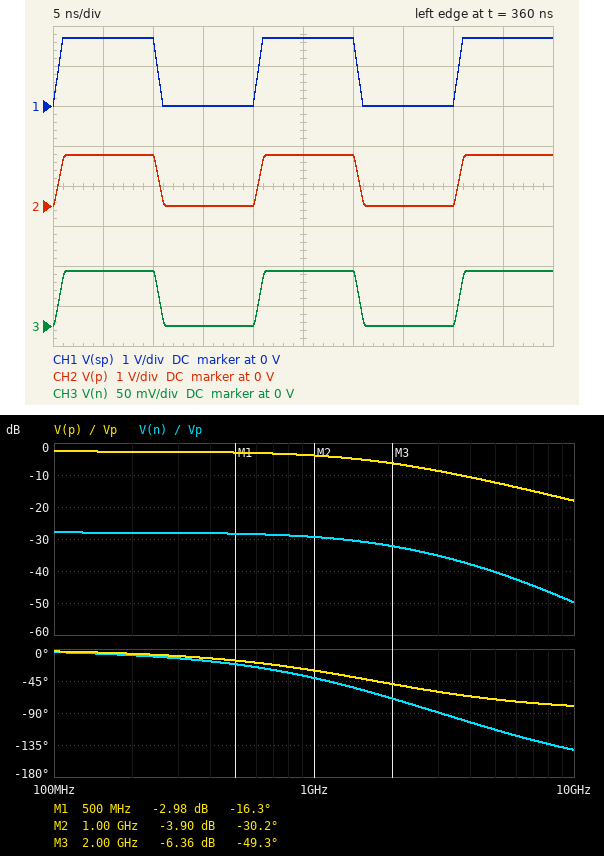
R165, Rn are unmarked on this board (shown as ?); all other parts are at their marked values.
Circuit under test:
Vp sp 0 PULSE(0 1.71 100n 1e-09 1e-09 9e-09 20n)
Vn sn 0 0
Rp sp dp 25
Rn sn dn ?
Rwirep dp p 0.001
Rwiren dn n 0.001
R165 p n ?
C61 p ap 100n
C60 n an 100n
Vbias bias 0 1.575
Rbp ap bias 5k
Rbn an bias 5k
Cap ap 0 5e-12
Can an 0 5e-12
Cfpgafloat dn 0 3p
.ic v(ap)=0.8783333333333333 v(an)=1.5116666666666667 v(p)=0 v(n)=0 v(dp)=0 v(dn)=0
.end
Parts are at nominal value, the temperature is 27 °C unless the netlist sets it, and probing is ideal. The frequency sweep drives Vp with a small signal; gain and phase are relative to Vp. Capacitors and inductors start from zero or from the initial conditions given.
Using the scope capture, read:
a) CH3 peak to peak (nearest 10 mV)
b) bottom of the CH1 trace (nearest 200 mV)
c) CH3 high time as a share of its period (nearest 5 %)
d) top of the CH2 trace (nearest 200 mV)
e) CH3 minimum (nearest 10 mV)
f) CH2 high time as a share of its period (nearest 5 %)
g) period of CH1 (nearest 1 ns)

70 mV
0 V
50 %
1.2 V
0 V
50 %
20 ns
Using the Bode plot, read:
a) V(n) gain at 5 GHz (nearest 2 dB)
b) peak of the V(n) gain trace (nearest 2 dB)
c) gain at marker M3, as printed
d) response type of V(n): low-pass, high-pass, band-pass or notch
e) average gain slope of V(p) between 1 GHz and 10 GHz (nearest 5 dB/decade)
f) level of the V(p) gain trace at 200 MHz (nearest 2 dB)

-40 dB
-28 dB
-6.36 dB
low-pass
-15 dB/decade
-2 dB
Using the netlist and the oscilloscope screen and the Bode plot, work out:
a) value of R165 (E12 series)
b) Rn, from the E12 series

68 Ω
3.9 Ω
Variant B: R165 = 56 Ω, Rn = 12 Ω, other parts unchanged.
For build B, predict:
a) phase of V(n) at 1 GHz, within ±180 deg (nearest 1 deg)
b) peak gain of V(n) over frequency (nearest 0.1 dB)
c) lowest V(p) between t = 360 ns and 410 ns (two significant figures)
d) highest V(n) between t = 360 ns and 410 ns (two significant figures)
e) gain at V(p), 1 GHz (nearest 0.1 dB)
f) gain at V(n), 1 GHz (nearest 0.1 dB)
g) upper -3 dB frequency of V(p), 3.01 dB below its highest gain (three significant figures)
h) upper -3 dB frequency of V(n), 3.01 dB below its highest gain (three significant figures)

-57 deg
-17.8 dB
2.6 mV
220 mV
-4.1 dB
-20.2 dB
1.66 GHz
1.16 GHz
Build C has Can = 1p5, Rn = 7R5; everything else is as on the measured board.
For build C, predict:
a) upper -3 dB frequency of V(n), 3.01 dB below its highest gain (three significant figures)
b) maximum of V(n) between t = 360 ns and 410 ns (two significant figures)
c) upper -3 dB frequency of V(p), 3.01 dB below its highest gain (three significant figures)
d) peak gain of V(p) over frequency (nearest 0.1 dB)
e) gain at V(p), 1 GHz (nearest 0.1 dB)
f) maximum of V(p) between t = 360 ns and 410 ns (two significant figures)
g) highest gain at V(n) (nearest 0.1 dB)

1.54 GHz
130 mV
1.68 GHz
-2.5 dB
-3.8 dB
1.3 V
-22.6 dB
